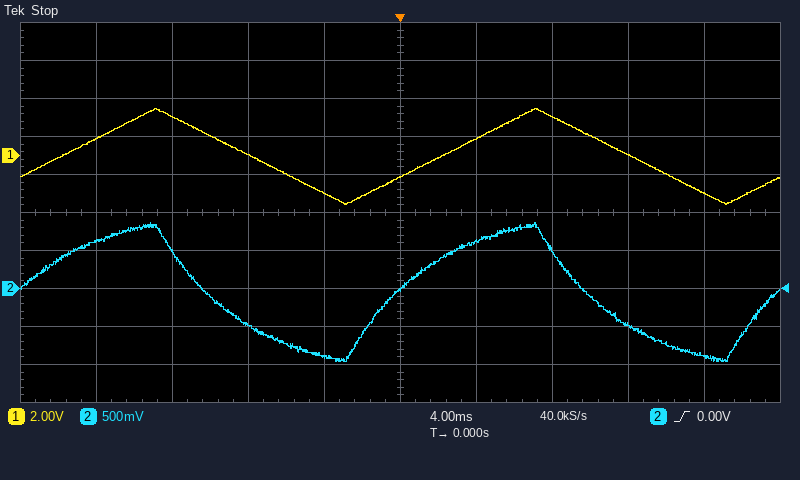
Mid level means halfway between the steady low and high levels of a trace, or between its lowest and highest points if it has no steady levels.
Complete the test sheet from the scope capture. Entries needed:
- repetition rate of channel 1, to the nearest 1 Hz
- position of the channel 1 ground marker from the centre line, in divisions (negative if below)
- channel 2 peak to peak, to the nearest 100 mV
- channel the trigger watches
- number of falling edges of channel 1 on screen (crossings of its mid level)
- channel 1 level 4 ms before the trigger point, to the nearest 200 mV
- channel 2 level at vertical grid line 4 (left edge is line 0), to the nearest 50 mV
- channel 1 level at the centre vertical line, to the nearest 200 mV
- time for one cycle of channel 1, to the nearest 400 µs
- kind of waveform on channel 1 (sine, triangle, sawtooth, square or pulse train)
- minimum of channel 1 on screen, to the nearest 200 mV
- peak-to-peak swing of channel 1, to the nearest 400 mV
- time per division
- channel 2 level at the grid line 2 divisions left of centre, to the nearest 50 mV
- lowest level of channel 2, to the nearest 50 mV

50 Hz
+1.5 div
1.80 V
channel 2
2
-2.0 V
-900 mV
-1.2 V
20.0 ms
triangle
-2.6 V
5.2 V
4 ms
-500 mV
-950 mV
